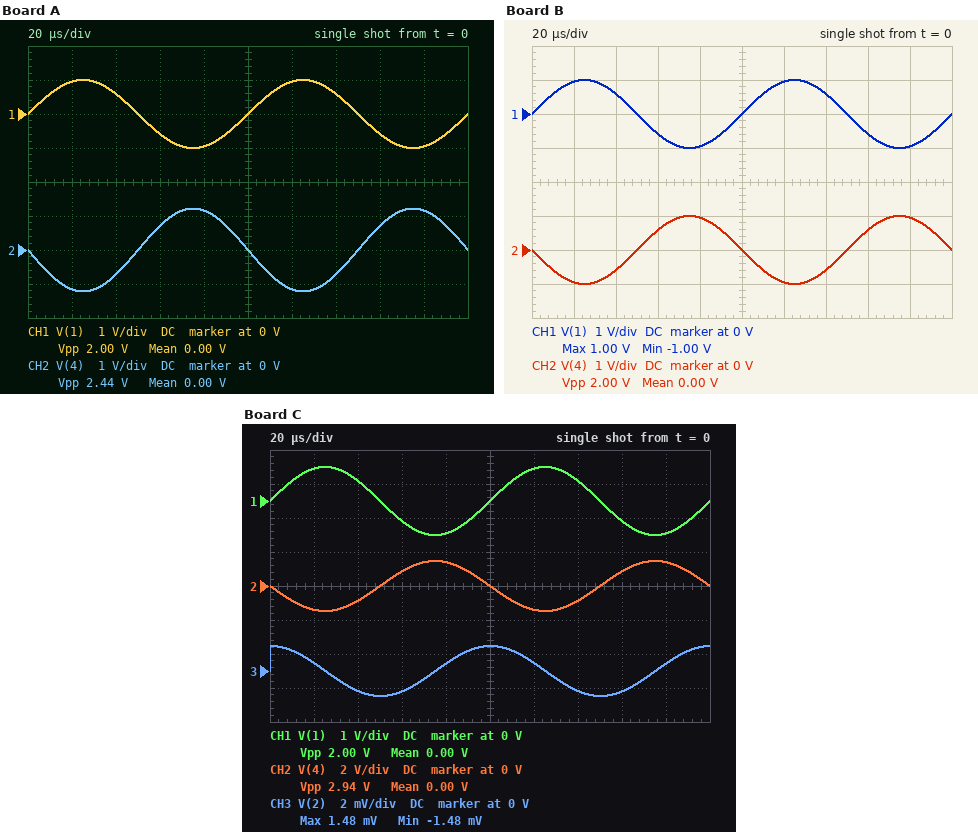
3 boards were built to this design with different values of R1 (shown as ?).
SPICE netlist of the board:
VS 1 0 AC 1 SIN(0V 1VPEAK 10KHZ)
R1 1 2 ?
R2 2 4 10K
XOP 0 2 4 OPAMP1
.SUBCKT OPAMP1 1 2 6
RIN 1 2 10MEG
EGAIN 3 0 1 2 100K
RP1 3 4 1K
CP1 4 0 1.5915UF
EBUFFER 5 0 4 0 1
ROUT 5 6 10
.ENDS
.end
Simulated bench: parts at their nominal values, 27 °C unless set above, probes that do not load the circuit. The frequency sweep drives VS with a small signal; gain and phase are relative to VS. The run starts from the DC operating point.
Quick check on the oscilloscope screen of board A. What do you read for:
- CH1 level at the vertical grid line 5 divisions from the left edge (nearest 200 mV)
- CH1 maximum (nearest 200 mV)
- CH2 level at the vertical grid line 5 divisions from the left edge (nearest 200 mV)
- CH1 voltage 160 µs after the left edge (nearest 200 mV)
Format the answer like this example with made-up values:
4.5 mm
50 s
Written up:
0 V
1.0 V
0 V
-600 mV
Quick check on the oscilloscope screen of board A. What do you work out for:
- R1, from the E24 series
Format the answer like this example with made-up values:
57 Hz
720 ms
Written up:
8.2 kΩ
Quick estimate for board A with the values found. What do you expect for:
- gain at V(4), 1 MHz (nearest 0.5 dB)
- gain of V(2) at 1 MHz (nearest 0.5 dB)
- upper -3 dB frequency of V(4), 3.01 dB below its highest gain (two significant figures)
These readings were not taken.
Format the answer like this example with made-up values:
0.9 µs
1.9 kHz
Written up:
1.5 dB
-18.5 dB
4.5 MHz
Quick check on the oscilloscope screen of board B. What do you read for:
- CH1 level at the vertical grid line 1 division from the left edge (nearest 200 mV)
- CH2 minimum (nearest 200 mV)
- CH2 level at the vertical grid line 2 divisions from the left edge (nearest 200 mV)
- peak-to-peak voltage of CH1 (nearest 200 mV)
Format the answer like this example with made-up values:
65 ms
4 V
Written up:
1.0 V
-1.0 V
-600 mV
2.0 V
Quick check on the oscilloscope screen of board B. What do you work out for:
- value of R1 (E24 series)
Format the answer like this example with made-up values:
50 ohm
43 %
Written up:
10 kΩ
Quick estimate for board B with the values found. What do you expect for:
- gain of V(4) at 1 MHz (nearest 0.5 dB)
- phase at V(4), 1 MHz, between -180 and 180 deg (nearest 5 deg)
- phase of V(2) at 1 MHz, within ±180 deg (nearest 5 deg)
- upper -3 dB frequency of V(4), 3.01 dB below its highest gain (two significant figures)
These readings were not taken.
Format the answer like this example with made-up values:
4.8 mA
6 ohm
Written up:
0 dB
170 deg
80 deg
5.0 MHz
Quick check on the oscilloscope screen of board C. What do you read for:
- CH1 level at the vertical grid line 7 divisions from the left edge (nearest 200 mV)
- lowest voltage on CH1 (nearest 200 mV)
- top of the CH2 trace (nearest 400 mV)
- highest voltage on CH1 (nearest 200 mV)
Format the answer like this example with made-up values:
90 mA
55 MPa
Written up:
600 mV
-1.0 V
1.6 V
1.0 V
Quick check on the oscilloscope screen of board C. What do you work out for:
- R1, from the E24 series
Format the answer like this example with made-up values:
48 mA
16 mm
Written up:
6.8 kΩ
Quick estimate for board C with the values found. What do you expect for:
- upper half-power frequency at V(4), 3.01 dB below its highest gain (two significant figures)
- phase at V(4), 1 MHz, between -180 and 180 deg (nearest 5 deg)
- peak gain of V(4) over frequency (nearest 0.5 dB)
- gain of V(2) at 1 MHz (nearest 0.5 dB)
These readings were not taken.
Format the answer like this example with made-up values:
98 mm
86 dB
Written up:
4.0 MHz
165 deg
3.5 dB
-17.0 dB
